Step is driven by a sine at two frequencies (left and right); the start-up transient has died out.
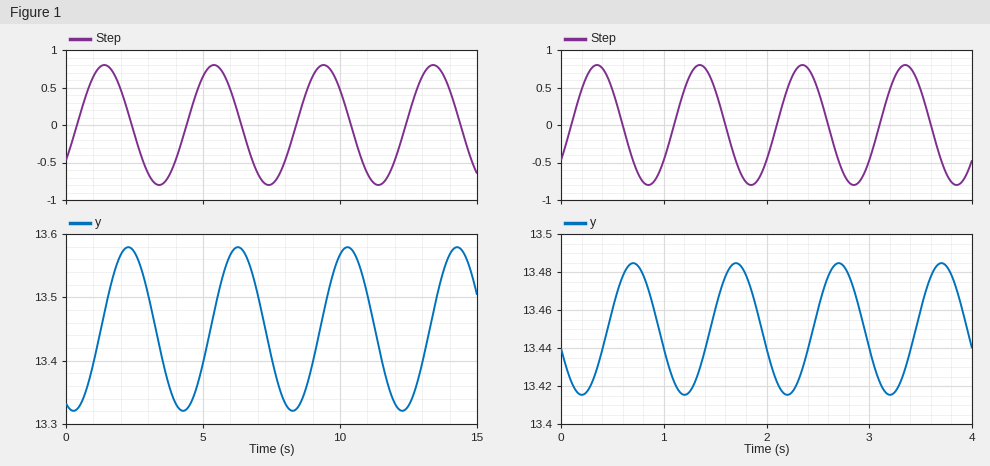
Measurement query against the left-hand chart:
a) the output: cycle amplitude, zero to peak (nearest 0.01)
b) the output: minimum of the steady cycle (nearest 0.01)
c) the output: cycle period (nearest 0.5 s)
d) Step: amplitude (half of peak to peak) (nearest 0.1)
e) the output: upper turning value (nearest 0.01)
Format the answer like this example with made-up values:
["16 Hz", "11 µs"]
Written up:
["0.13", "13.32", "4.0 s", "0.8", "13.58"]
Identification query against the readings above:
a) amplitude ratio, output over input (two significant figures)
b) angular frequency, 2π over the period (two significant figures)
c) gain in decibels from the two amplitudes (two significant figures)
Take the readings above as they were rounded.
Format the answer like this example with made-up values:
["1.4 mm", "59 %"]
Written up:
["0.16", "1.6 rad/s", "-16 dB"]
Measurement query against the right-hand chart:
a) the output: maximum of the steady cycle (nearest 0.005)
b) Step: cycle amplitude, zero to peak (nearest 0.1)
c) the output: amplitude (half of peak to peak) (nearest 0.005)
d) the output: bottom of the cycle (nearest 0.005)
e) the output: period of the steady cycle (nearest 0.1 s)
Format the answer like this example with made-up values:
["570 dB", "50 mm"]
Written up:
["13.485", "0.8", "0.035", "13.415", "1.0 s"]
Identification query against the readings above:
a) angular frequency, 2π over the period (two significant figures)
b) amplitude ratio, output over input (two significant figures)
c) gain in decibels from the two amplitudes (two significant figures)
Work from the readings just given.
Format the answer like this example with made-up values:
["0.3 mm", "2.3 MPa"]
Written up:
["6.3 rad/s", "0.044", "-27 dB"]
